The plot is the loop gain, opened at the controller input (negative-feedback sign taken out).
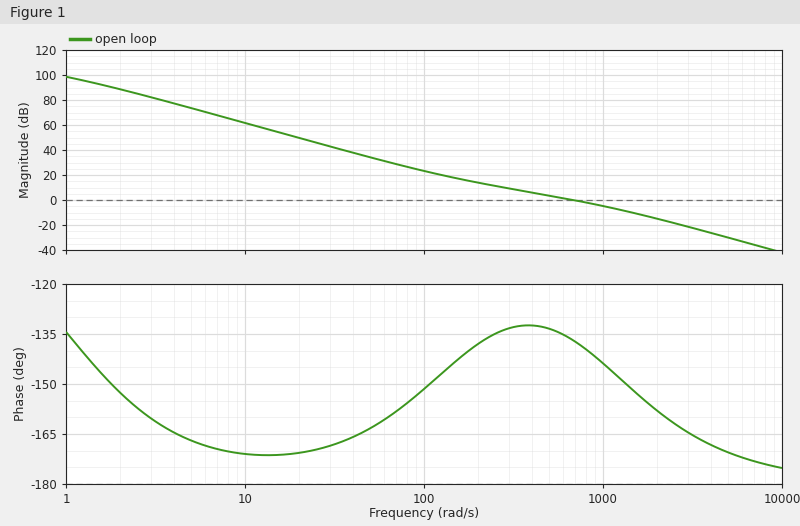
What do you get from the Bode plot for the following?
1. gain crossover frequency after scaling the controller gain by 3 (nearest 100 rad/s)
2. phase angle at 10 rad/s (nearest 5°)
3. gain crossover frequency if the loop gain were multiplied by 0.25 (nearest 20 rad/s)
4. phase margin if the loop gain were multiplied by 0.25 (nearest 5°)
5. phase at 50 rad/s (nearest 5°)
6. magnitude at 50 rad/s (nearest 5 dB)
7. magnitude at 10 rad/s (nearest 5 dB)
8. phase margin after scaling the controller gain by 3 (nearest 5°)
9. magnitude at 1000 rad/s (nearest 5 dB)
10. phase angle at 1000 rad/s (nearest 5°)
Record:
1400 rad/s
-170°
240 rad/s
45°
-165°
35 dB
60 dB
30°
-5 dB
-145°
